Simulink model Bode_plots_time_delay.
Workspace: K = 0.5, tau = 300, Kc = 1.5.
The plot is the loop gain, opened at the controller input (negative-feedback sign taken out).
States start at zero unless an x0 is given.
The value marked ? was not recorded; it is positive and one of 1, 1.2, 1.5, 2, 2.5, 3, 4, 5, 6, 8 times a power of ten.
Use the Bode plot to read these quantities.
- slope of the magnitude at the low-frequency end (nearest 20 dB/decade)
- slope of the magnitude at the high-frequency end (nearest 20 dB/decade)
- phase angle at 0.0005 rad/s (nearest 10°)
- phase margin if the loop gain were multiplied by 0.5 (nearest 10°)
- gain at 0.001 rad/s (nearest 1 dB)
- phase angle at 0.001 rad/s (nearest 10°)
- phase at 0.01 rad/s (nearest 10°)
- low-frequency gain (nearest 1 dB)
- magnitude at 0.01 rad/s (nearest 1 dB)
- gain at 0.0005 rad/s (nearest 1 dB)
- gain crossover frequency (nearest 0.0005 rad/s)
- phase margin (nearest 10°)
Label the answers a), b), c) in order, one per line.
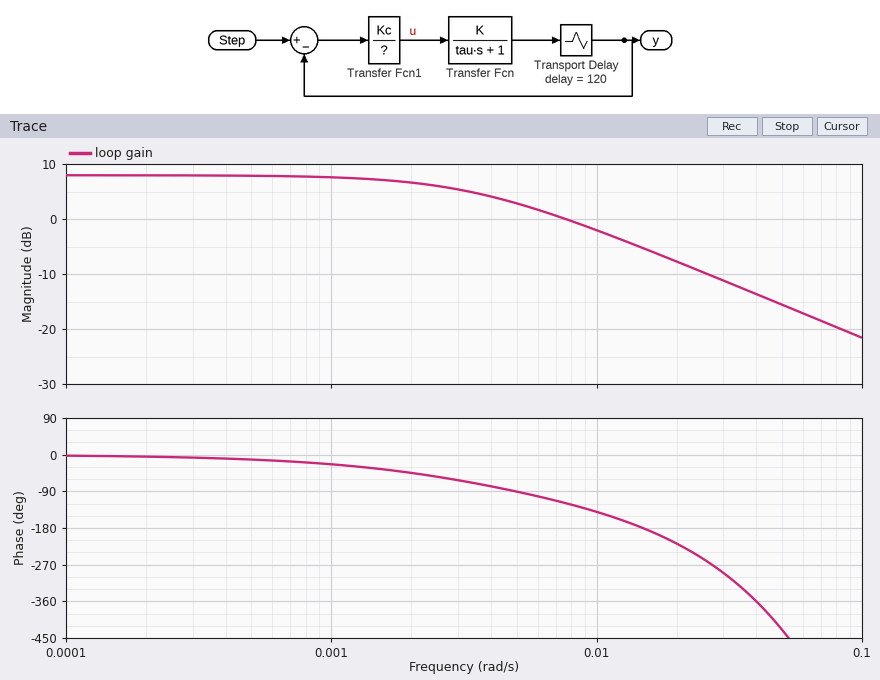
a) 0 dB/decade
b) -20 dB/decade
c) -10°
d) 130°
e) 8 dB
f) -20°
g) -140°
h) 8 dB
i) -2 dB
j) 8 dB
k) 0.0075 rad/s
l) 60°
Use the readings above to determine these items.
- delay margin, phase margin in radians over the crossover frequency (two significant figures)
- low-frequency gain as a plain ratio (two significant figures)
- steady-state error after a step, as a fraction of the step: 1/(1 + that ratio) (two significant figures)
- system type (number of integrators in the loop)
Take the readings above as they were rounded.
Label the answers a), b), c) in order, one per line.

a) 140 s
b) 2.5
c) 0.29
d) 0
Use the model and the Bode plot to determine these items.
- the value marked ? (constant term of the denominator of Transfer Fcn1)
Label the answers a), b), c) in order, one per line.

a) 0.3
